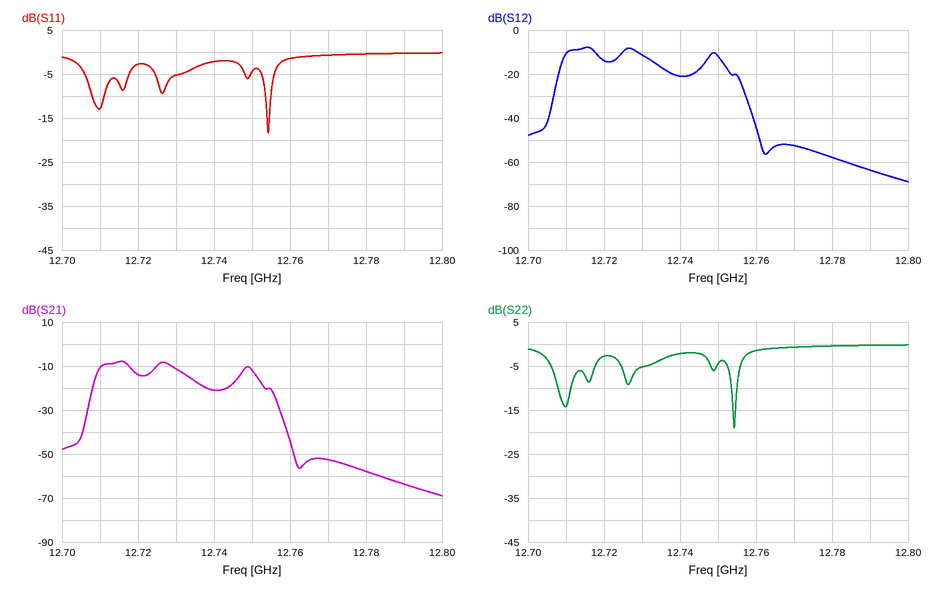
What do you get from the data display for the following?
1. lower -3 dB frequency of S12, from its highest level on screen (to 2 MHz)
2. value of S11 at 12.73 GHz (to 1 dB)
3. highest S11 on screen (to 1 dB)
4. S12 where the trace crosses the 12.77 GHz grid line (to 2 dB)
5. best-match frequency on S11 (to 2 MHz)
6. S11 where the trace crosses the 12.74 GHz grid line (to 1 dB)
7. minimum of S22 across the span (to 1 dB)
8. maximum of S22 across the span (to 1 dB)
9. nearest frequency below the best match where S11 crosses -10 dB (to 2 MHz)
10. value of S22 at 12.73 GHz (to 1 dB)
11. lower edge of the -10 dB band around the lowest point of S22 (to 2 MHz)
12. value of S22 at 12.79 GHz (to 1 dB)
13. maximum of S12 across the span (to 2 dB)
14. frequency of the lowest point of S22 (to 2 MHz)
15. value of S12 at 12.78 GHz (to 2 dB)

12.710 GHz
-5 dB
0 dB
-52 dB
12.754 GHz
-2 dB
-19 dB
0 dB
12.754 GHz
-5 dB
12.754 GHz
0 dB
-8 dB
12.754 GHz
-58 dB
